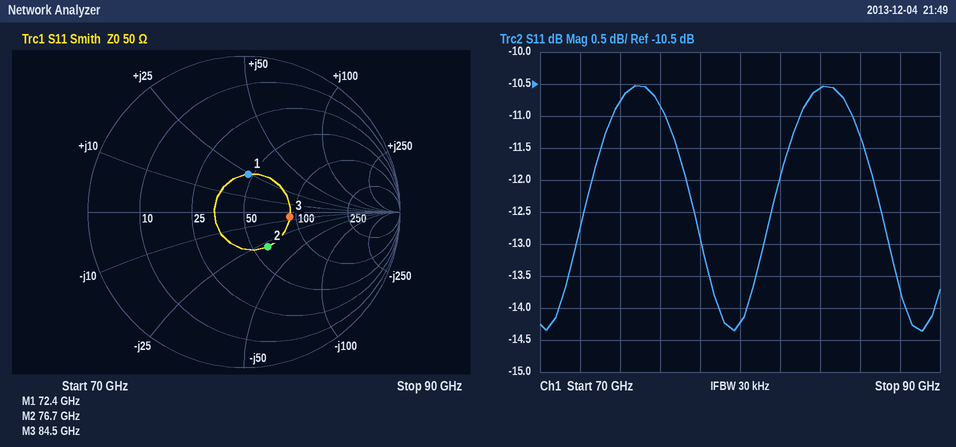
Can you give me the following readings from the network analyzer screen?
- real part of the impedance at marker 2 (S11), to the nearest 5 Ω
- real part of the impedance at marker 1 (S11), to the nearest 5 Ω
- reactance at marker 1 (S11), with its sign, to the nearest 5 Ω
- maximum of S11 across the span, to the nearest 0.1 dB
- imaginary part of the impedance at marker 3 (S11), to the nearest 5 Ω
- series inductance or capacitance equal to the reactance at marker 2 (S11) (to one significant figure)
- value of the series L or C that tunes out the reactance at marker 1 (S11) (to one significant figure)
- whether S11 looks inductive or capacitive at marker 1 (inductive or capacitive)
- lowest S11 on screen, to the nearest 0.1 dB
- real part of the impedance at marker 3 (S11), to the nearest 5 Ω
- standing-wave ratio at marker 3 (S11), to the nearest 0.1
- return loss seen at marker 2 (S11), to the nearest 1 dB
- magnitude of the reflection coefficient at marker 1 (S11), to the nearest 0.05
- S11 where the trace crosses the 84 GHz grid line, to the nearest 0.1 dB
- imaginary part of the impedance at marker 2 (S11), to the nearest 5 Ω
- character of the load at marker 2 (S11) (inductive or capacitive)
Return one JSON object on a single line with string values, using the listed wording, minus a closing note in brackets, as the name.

{"real part of the impedance at marker 2 (S11), to the nearest 5 Ω": "60 Ω", "real part of the impedance at marker 1 (S11), to the nearest 5 Ω": "45 Ω", "reactance at marker 1 (S11), with its sign, to the nearest 5 Ω": "+25 Ω", "maximum of S11 across the span, to the nearest 0.1 dB": "-10.5 dB", "imaginary part of the impedance at marker 3 (S11), to the nearest 5 Ω": "-5 Ω", "series inductance or capacitance equal to the reactance at marker 2 (S11)": "70 fF", "value of the series L or C that tunes out the reactance at marker 1 (S11)": "90 fF", "whether S11 looks inductive or capacitive at marker 1": "inductive", "lowest S11 on screen, to the nearest 0.1 dB": "-14.4 dB", "real part of the impedance at marker 3 (S11), to the nearest 5 Ω": "90 Ω", "standing-wave ratio at marker 3 (S11), to the nearest 0.1": "1.8", "return loss seen at marker 2 (S11), to the nearest 1 dB": "11 dB", "magnitude of the reflection coefficient at marker 1 (S11), to the nearest 0.05": "0.25", "S11 where the trace crosses the 84 GHz grid line, to the nearest 0.1 dB": "-10.6 dB", "imaginary part of the impedance at marker 2 (S11), to the nearest 5 Ω": "-30 Ω", "character of the load at marker 2 (S11)": "capacitive"}
